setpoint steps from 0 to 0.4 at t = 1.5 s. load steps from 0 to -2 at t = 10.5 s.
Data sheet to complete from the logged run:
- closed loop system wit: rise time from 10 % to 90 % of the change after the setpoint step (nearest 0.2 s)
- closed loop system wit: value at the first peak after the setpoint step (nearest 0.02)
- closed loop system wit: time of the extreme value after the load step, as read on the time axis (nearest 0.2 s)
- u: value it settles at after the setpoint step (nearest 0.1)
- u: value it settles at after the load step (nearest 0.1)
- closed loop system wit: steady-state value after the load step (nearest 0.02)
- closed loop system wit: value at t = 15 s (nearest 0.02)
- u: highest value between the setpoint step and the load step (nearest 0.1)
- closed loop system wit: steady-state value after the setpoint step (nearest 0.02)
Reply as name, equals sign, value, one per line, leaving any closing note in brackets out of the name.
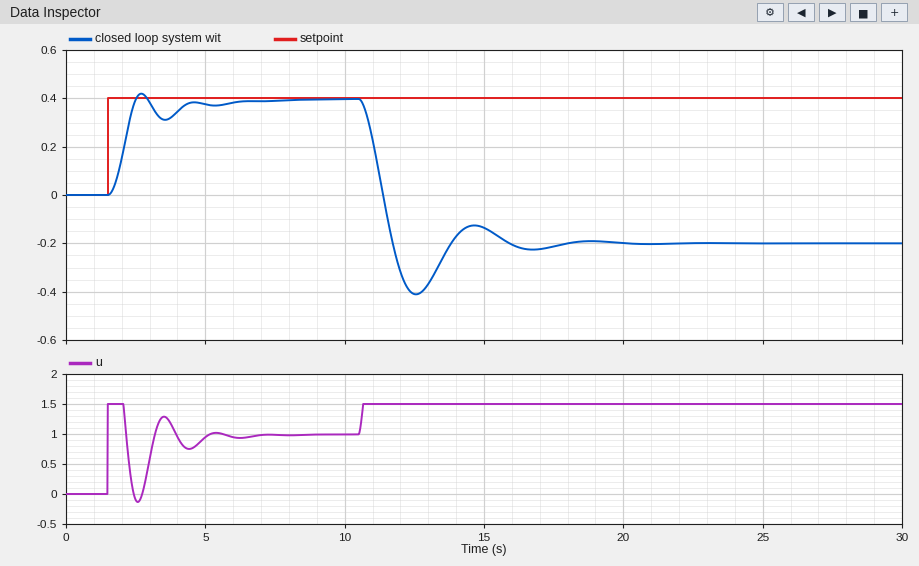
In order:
closed loop system wit: rise time from 10 % to 90 % of the change after the setpoint step = 0.6 s
closed loop system wit: value at the first peak after the setpoint step = 0.42
closed loop system wit: time of the extreme value after the load step, as read on the time axis = 12.6 s
u: value it settles at after the setpoint step = 1.0
u: value it settles at after the load step = 1.5
closed loop system wit: steady-state value after the load step = -0.20
closed loop system wit: value at t = 15 s = -0.14
u: highest value between the setpoint step and the load step = 1.5
closed loop system wit: steady-state value after the setpoint step = 0.40
